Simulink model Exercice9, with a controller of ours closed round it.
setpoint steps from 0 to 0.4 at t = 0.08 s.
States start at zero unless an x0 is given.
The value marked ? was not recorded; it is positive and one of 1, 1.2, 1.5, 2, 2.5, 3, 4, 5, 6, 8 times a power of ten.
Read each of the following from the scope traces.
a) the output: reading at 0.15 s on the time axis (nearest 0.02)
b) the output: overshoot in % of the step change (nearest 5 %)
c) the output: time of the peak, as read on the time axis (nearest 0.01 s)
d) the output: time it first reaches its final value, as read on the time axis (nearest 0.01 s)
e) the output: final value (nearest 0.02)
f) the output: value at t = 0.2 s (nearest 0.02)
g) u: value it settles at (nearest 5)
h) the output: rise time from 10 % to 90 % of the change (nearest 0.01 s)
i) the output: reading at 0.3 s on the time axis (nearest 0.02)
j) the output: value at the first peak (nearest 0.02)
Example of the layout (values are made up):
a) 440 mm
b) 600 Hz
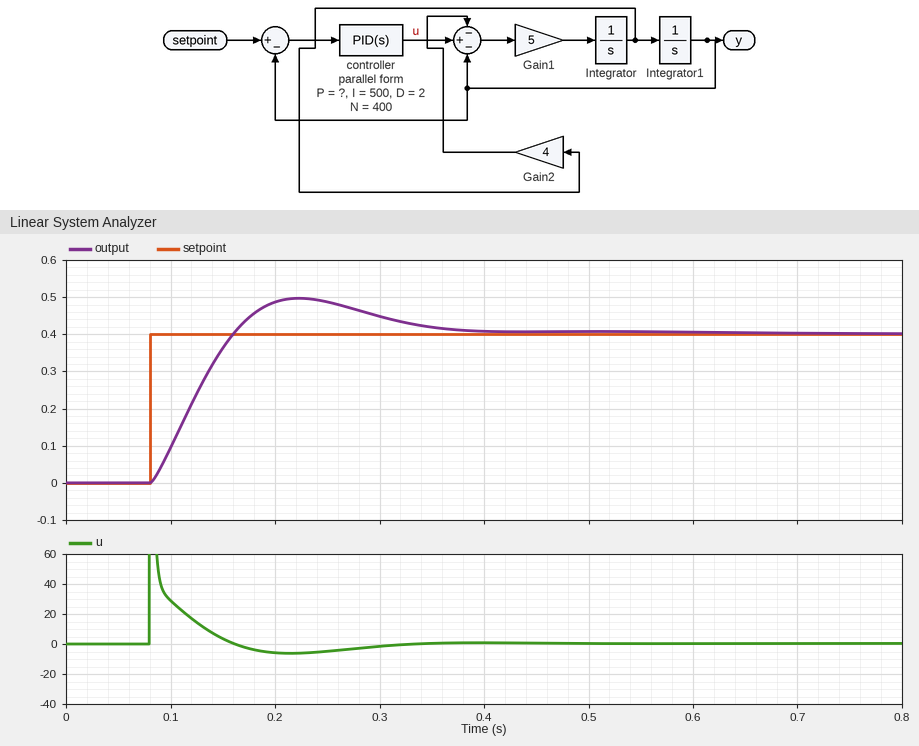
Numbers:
a) 0.36
b) 25 %
c) 0.22 s
d) 0.16 s
e) 0.40
f) 0.48
g) 0
h) 0.06 s
i) 0.44
j) 0.50
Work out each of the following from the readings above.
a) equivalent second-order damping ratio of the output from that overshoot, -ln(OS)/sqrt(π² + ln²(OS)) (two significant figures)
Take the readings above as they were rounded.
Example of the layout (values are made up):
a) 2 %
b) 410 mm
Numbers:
a) 0.40
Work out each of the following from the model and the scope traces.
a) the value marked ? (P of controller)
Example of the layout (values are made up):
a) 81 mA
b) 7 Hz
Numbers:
a) 120
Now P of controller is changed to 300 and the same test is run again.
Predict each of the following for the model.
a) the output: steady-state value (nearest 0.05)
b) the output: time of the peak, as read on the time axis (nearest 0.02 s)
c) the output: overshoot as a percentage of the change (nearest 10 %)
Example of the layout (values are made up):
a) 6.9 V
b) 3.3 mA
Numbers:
a) 0.40
b) 0.16 s
c) 30 %
